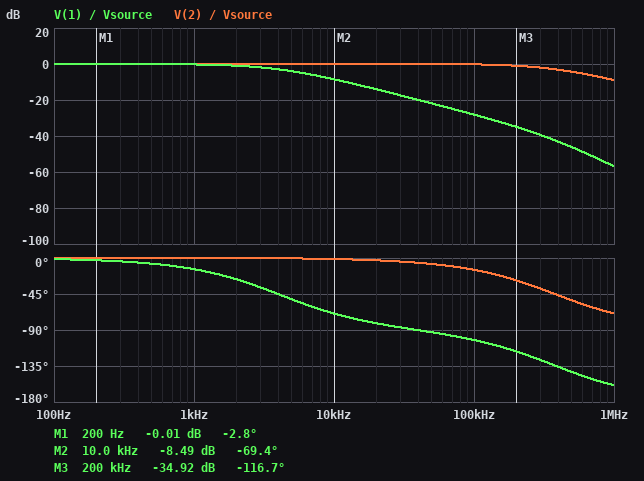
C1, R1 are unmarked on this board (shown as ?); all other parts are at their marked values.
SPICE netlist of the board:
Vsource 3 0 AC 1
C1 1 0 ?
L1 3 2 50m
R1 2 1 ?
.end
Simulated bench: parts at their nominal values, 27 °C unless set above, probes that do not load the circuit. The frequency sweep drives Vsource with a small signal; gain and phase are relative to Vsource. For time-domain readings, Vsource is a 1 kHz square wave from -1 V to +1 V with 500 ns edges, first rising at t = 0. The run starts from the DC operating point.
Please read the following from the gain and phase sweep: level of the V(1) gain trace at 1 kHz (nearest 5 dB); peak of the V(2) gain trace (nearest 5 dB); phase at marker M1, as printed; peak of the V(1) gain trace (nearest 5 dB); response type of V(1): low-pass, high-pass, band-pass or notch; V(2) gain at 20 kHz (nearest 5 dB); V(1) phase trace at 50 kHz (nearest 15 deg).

0 dB
0 dB
-2.8 deg
0 dB
low-pass
0 dB
-90 deg
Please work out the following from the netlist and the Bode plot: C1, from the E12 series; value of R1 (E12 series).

330 pF
120 kΩ
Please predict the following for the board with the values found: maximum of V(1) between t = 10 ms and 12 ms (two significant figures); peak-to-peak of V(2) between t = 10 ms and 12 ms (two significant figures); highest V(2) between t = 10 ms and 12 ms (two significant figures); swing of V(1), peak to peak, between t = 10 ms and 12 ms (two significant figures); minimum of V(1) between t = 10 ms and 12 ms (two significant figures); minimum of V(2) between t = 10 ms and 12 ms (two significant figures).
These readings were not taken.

1.0 V
2.0 V
1.0 V
2.0 V
-1.0 V
-1.0 V
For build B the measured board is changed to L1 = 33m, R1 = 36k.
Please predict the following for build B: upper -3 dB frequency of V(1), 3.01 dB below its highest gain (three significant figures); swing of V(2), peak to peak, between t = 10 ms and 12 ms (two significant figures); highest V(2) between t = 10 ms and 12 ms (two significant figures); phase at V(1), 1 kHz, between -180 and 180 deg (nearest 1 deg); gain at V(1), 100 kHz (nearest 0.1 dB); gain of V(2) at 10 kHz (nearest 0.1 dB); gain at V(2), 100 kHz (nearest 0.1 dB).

14.5 kHz
2.2 V
1.1 V
-4 deg
-18.2 dB
0.2 dB
-0.7 dB
